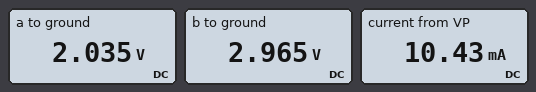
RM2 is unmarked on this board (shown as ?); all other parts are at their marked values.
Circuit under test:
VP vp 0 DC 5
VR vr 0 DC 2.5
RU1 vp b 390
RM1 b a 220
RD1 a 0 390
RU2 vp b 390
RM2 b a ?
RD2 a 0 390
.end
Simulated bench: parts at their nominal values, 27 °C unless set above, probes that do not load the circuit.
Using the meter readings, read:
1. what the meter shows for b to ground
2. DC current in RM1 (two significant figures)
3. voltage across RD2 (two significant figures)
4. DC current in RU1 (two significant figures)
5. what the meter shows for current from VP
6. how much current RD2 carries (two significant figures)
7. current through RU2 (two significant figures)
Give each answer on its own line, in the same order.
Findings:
2.965 V
4.2 mA
2.0 V
5.2 mA
10.43 mA
5.2 mA
5.2 mA
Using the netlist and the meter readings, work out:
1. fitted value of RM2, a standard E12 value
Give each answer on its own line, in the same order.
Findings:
150 Ω
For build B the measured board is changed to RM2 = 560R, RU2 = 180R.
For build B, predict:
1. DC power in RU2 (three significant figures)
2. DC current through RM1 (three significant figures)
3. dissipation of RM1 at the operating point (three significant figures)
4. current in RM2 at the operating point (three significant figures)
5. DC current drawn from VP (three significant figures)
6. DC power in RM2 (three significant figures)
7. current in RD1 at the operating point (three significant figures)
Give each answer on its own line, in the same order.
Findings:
9.29 mW
7.54 mA
12.5 mW
2.96 mA
10.5 mA
4.91 mW
5.25 mA
